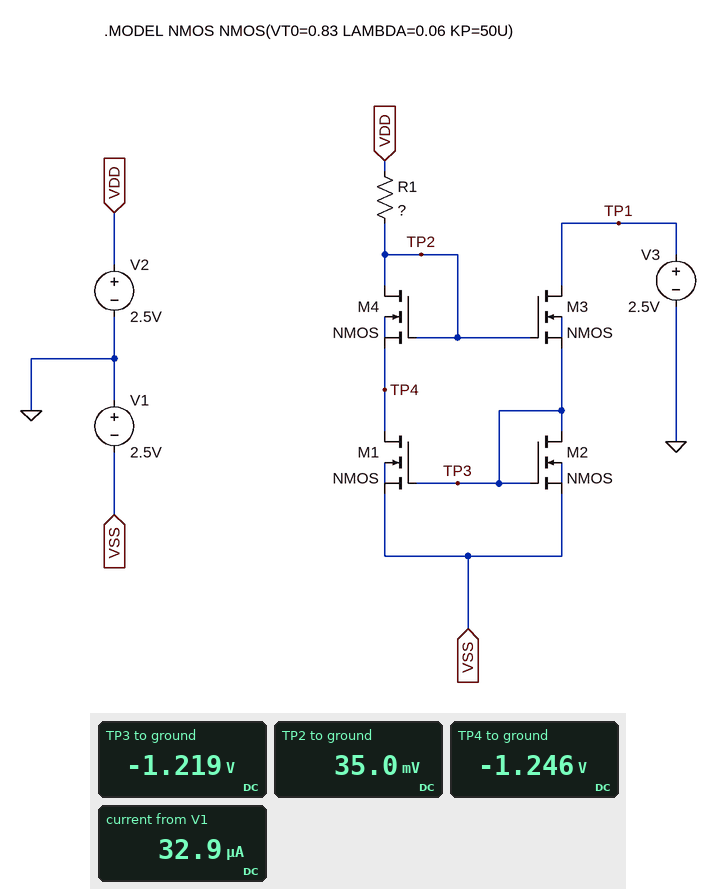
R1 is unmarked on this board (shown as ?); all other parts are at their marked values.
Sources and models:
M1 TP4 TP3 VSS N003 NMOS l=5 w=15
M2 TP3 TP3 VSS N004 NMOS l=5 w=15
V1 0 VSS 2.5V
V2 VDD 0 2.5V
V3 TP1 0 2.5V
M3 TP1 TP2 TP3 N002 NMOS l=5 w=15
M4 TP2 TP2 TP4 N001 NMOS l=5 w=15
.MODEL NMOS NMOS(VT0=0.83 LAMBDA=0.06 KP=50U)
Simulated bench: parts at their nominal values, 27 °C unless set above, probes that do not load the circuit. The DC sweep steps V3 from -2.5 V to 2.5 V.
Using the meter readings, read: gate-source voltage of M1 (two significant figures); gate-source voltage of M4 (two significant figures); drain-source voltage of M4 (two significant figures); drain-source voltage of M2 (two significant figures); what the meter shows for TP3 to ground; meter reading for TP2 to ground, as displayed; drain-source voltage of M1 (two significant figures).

1.3 V
1.3 V
1.3 V
1.3 V
-1.219 V
35.0 mV
1.3 V
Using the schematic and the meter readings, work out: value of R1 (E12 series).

150 kΩ
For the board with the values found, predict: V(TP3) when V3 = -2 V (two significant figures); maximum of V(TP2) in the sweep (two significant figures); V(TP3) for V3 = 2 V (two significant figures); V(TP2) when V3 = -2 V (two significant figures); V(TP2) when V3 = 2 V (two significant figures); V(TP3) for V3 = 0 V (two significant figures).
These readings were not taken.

-2.0 V
2.5 V
-1.2 V
2.5 V
39 mV
-1.2 V
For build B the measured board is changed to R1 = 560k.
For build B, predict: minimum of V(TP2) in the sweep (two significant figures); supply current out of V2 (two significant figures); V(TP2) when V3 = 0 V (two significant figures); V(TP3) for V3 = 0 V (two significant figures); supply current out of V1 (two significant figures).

-350 mV
5.1 µA
-340 mV
-1.4 V
10 µA
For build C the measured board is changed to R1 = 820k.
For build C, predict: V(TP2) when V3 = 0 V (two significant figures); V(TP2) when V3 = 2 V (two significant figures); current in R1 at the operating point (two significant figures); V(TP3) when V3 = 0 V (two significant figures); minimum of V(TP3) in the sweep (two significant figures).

-420 mV
-430 mV
3.6 µA
-1.5 V
-2.5 V
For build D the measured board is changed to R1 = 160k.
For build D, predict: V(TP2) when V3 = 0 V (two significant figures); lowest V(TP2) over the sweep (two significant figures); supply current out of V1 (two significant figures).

34 mV
11 mV
31 µA
